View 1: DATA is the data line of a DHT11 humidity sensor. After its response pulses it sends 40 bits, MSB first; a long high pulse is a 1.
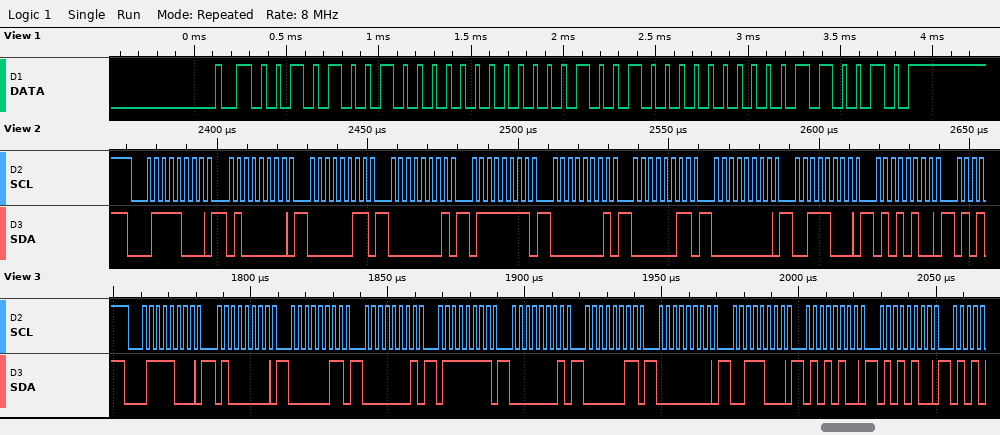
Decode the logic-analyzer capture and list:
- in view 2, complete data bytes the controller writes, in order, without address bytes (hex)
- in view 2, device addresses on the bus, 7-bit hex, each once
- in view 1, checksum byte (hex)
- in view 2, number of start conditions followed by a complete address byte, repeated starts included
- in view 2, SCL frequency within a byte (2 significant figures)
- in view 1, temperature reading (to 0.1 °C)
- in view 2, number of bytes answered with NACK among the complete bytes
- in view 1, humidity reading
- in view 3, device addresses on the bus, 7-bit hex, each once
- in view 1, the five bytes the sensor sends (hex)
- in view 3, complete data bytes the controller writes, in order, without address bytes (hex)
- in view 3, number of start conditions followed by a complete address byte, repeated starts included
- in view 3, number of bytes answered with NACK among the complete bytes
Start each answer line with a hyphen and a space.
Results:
- 40 03 01 7F 01 03 00 38 54
- 0x3C
- 0x32
- 1
- 400 kHz
- 9.0 °C
- 0
- 41 %
- 0x3C
- 29 00 09 00 32
- 40 03 01 7F 01 03 00 38 54 54
- 1
- 0
